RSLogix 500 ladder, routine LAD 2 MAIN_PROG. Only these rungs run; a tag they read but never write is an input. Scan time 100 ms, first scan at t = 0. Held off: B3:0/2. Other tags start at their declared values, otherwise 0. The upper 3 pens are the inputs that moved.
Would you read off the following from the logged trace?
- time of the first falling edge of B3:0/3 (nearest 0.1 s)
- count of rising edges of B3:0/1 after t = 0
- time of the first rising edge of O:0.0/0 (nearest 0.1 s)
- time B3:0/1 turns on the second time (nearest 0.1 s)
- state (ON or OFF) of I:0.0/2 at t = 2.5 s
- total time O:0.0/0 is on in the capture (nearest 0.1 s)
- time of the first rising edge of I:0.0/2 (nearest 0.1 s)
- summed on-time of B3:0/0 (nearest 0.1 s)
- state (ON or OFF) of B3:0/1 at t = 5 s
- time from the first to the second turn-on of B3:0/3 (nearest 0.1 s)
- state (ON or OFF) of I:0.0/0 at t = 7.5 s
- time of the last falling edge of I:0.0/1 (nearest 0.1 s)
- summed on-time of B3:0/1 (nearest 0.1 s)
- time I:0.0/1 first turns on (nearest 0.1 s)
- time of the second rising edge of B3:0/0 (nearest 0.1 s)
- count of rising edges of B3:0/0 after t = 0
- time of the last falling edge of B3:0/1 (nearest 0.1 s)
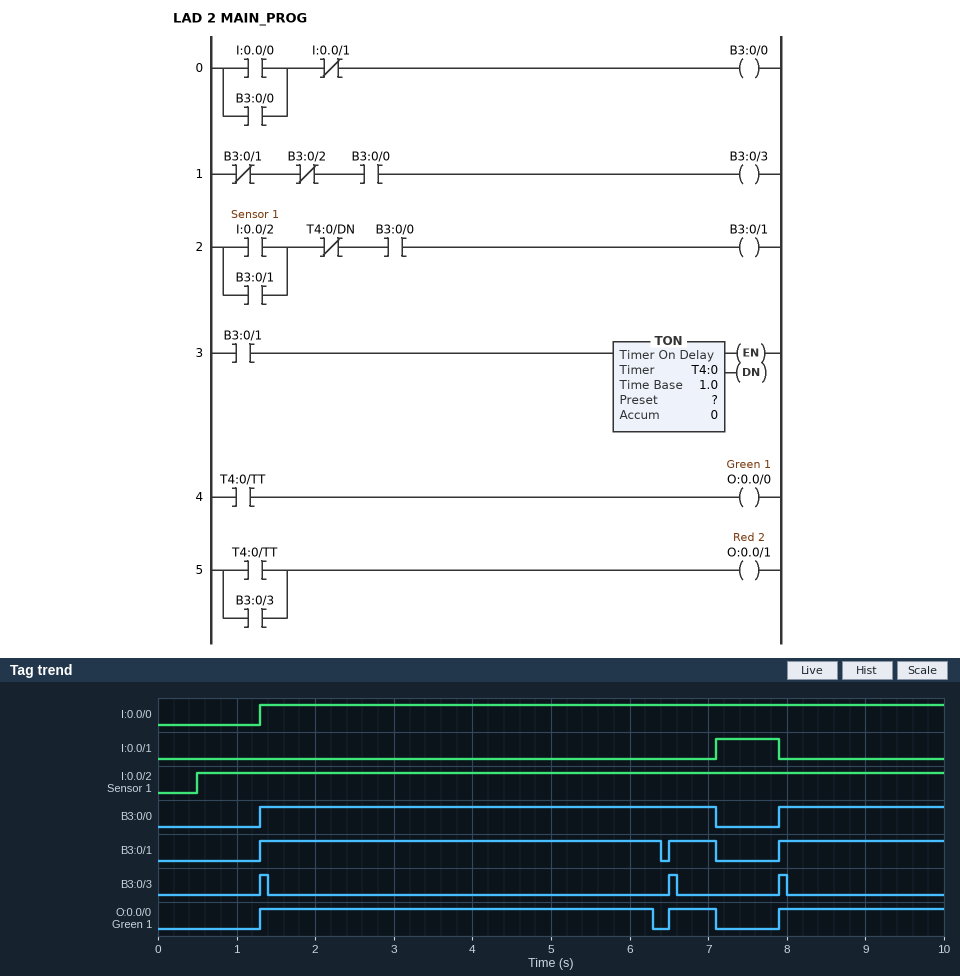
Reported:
1.4 s
3
1.3 s
6.5 s
ON
7.7 s
0.5 s
7.9 s
ON
5.2 s
ON
7.9 s
7.8 s
7.1 s
7.9 s
2
7.1 s
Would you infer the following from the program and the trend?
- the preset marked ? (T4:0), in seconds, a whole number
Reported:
5 s
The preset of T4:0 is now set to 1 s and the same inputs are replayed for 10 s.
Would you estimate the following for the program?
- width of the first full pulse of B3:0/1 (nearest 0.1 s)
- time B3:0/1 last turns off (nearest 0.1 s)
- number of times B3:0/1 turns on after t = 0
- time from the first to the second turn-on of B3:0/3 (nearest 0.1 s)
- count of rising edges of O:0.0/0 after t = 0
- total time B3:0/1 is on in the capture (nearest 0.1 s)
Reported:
1.1 s
9.0 s
7
1.2 s
7
7.4 s
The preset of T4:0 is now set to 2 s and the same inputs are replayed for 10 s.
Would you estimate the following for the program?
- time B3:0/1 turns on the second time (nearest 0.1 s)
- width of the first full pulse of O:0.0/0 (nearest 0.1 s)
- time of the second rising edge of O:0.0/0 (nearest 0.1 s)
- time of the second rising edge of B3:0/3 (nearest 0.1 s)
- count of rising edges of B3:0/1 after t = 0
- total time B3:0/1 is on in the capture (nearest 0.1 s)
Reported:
3.5 s
2.0 s
3.5 s
3.5 s
4
7.7 s
